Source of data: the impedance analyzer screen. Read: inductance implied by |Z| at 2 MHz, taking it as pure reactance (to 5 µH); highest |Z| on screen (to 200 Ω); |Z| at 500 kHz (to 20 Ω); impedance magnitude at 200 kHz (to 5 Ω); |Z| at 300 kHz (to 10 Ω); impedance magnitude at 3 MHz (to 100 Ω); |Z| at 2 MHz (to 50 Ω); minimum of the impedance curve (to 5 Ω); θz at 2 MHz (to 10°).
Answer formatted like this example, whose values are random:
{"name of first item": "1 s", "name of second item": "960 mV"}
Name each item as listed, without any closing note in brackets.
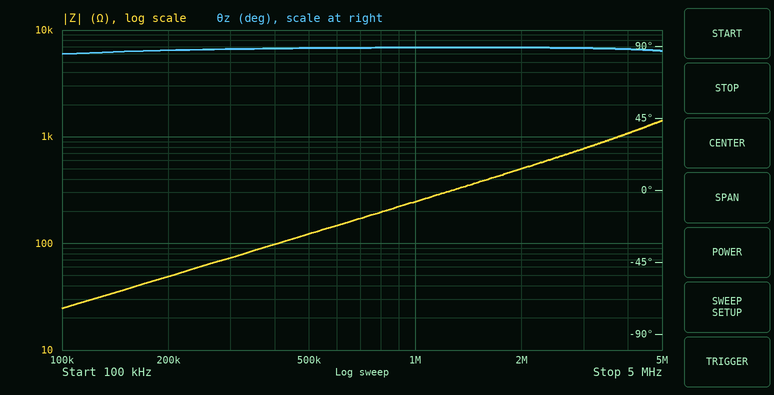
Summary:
{"inductance implied by |Z| at 2 MHz, taking it as pure reactance": "40 µH", "highest |Z| on screen": "1.4 kΩ", "|Z| at 500 kHz": "120 Ω", "impedance magnitude at 200 kHz": "50 Ω", "|Z| at 300 kHz": "70 Ω", "impedance magnitude at 3 MHz": "800 Ω", "|Z| at 2 MHz": "500 Ω", "minimum of the impedance curve": "25 Ω", "θz at 2 MHz": "90°"}
